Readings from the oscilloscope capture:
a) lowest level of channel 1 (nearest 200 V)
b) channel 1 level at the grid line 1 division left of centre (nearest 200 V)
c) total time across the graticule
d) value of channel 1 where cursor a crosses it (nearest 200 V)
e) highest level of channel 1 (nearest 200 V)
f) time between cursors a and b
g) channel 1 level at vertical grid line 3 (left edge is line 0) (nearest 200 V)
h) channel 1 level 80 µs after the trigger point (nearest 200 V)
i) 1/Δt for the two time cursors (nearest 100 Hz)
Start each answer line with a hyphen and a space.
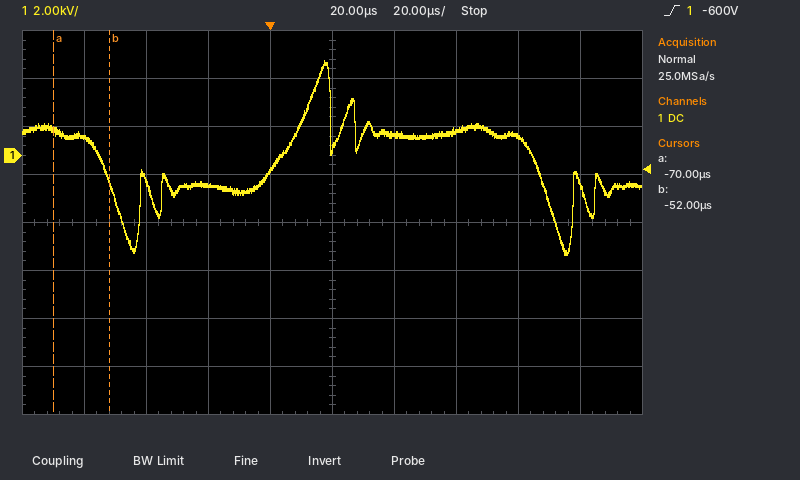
- -4.2 kV
- -600 V
- 200 µs
- 1.0 kV
- 4.0 kV
- 18 µs
- -1.2 kV
- 800 V
- 55.6 kHz
